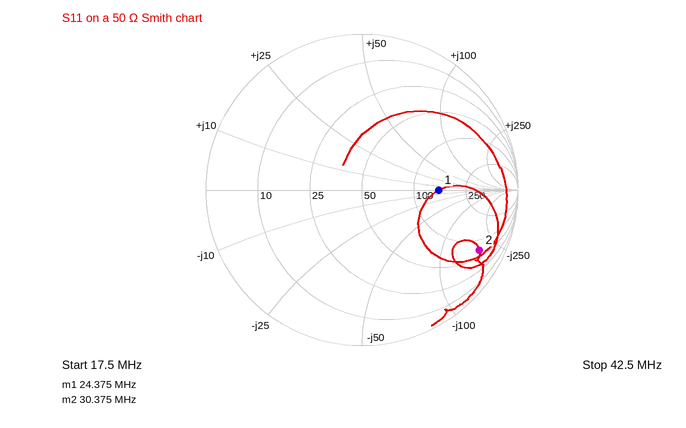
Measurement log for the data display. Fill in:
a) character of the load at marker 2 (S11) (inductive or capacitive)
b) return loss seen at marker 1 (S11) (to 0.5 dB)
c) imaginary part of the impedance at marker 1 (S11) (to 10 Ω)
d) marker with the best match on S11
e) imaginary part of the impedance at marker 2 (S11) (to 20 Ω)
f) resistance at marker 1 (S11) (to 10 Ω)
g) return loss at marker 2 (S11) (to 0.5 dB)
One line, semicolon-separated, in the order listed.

capacitive; 6.0 dB; 0 Ω; marker 1; -180 Ω; 150 Ω; 1.5 dB
